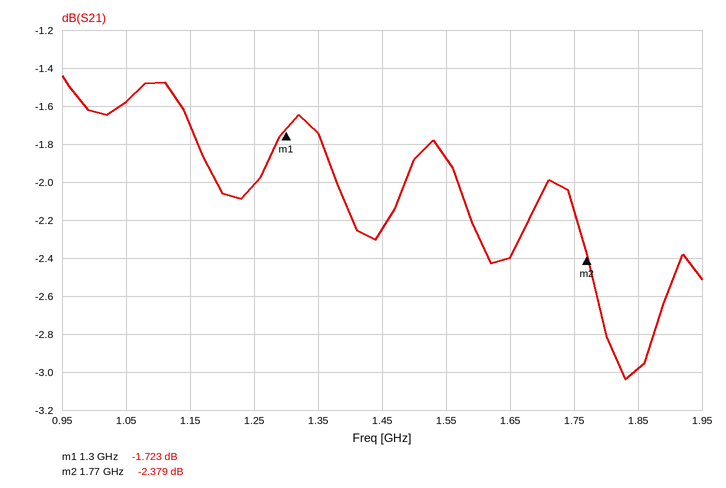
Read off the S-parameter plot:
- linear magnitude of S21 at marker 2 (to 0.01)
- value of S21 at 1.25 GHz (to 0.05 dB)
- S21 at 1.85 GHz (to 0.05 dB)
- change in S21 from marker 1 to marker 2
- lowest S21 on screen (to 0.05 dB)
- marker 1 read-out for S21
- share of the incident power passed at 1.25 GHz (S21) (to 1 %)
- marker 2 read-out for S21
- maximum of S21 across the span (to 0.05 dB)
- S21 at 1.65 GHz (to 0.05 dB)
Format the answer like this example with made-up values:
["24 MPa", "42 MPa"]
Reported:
["0.76", "-2.00 dB", "-3.00 dB", "-0.656 dB", "-3.05 dB", "-1.723 dB", "63 %", "-2.379 dB", "-1.45 dB", "-2.40 dB"]
